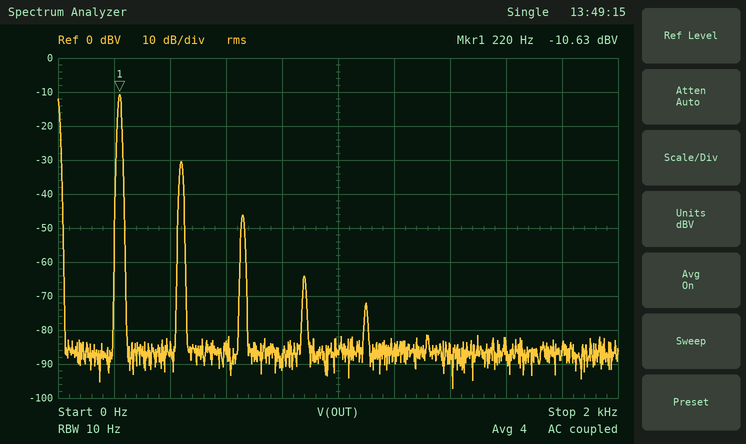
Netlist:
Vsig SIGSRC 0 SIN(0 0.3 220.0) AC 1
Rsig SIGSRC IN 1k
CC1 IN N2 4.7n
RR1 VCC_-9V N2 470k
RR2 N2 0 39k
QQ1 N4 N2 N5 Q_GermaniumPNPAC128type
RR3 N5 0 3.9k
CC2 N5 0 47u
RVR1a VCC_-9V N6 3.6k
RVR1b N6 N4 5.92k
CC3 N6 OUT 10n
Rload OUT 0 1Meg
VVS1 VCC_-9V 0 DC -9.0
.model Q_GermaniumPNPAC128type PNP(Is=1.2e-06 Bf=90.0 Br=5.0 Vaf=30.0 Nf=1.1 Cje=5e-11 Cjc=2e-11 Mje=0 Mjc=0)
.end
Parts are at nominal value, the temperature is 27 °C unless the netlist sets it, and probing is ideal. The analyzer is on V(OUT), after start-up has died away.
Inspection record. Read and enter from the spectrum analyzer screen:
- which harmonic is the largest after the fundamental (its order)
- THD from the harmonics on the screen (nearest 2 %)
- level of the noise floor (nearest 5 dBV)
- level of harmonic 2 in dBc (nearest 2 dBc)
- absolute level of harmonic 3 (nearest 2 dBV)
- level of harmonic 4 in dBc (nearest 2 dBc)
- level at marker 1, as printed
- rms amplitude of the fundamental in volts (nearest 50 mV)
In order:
2
10 %
-85 dBV
-20 dBc
-46 dBV
-54 dBc
-10.63 dBV
300 mV
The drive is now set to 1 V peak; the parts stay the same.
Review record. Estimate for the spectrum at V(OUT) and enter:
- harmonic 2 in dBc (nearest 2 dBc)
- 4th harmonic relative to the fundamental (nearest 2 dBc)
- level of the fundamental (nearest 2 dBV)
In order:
-8 dBc
-24 dBc
-4 dBV
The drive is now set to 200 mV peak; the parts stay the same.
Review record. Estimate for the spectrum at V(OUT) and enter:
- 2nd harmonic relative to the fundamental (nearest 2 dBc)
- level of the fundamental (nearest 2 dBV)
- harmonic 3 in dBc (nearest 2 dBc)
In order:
-24 dBc
-14 dBV
-42 dBc
